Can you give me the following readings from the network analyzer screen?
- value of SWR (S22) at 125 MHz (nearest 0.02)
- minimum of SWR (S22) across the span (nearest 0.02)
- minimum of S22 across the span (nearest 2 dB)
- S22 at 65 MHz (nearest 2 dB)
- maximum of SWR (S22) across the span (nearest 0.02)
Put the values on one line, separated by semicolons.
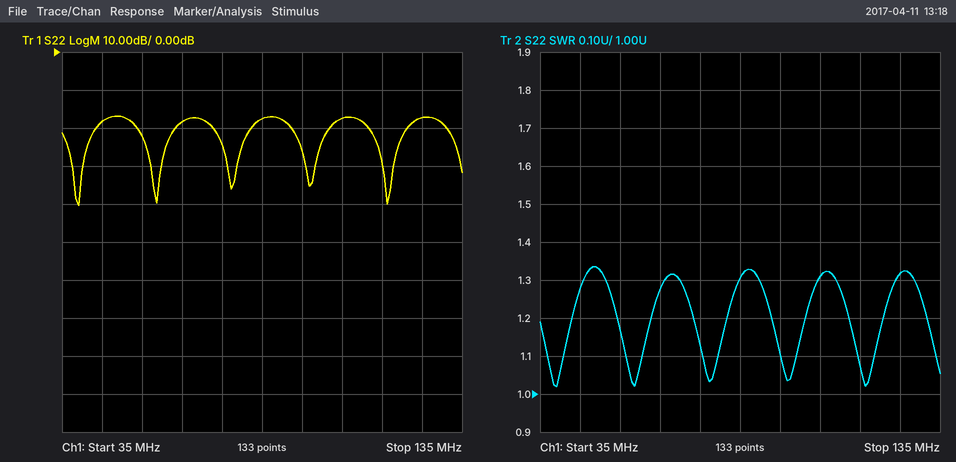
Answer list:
1.32; 1.02; -40 dB; -18 dB; 1.34
